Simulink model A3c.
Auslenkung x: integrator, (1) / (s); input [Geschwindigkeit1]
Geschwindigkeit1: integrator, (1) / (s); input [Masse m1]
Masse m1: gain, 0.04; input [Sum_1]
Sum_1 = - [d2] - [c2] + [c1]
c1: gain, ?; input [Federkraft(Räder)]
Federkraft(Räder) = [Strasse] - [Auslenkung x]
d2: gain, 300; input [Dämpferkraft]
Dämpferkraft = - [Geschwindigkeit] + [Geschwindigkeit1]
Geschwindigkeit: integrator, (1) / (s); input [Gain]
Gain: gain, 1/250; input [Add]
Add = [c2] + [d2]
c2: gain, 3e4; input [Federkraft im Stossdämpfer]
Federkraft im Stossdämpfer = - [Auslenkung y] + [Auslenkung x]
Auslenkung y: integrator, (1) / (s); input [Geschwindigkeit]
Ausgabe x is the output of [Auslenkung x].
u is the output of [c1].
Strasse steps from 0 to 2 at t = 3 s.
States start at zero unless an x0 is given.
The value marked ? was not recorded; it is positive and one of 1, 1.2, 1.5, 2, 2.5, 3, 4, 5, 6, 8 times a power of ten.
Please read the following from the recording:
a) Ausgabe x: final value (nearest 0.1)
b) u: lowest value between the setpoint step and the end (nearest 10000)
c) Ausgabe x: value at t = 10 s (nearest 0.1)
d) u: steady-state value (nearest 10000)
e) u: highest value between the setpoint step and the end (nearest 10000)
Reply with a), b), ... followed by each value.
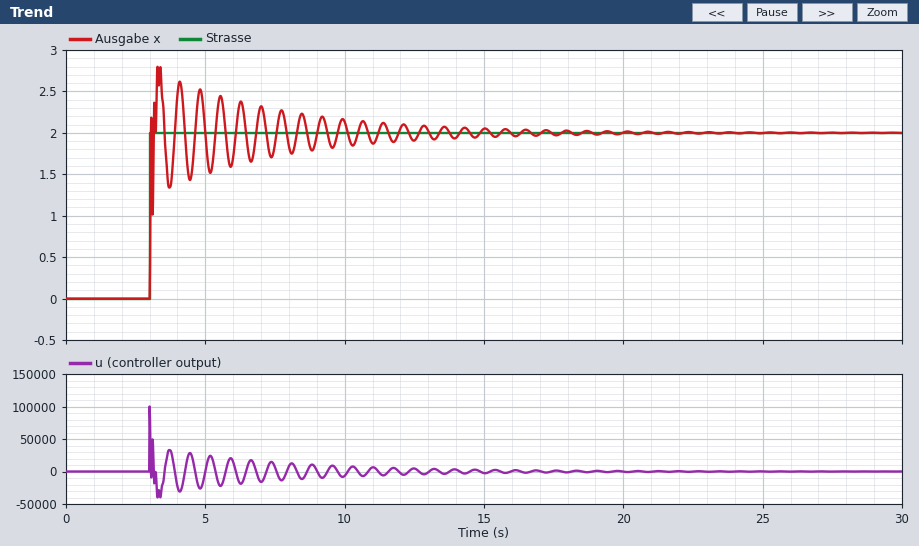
a) 2.0
b) -40000
c) 2.1
d) 0
e) 100000
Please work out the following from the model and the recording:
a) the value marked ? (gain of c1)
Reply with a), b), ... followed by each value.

a) 50000
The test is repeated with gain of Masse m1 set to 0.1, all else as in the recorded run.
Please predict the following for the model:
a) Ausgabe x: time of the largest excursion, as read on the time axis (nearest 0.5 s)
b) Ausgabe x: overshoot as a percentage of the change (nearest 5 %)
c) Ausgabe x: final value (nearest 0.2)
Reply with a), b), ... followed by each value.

a) 3.5 s
b) 35 %
c) 2.0
